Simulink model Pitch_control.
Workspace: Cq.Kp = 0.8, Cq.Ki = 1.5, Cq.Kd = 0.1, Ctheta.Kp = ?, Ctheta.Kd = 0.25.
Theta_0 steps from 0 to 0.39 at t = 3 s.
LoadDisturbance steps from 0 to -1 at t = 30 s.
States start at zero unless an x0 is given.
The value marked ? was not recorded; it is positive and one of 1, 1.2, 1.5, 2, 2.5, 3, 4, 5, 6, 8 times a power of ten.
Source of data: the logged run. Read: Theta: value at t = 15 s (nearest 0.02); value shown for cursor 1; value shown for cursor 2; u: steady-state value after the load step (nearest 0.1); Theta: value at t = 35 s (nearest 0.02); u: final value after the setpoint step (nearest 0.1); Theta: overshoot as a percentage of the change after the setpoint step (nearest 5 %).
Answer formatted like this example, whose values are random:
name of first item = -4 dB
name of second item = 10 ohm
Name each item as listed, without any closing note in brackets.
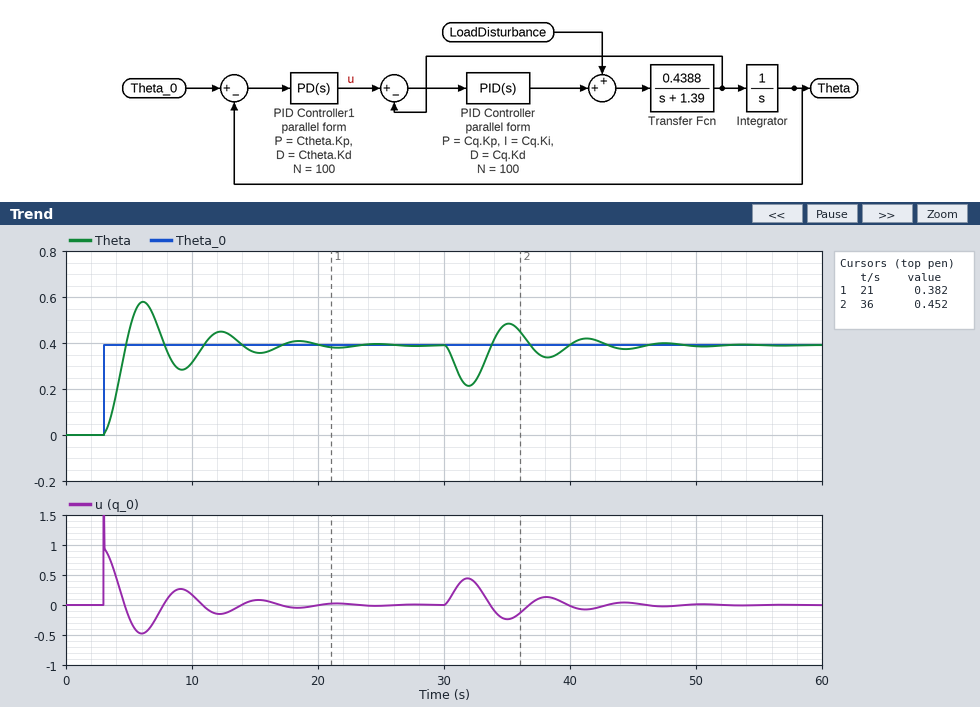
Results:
Theta: value at t = 15 s = 0.36
value shown for cursor 1 = 0.382
value shown for cursor 2 = 0.452
u: steady-state value after the load step = 0.0
Theta: value at t = 35 s = 0.48
u: final value after the setpoint step = 0.0
Theta: overshoot as a percentage of the change after the setpoint step = 50 %
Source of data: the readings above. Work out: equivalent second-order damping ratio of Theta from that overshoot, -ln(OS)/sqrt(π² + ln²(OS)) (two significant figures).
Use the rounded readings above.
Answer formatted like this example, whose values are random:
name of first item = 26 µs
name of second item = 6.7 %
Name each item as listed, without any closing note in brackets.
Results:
equivalent second-order damping ratio of Theta from that overshoot, -ln(OS)/sqrt(π² + ln²(OS)) = 0.22
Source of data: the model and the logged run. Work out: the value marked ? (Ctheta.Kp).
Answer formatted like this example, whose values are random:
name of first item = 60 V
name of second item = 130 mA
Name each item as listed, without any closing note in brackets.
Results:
the value marked ? = 2.5
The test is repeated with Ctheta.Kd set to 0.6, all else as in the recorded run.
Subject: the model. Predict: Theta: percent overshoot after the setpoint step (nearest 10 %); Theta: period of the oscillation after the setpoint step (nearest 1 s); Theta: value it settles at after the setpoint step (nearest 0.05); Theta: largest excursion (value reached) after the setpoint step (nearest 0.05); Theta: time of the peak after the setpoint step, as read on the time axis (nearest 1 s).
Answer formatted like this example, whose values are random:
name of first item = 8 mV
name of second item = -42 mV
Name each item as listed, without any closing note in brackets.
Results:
Theta: percent overshoot after the setpoint step = 40 %
Theta: period of the oscillation after the setpoint step = 6 s
Theta: value it settles at after the setpoint step = 0.40
Theta: largest excursion (value reached) after the setpoint step = 0.55
Theta: time of the peak after the setpoint step, as read on the time axis = 6 s
